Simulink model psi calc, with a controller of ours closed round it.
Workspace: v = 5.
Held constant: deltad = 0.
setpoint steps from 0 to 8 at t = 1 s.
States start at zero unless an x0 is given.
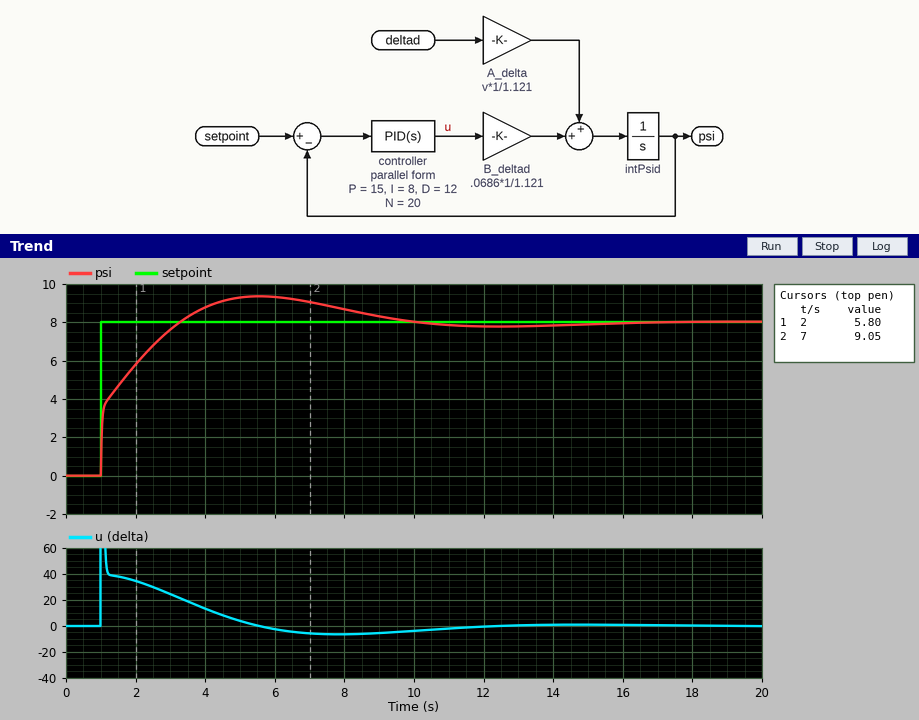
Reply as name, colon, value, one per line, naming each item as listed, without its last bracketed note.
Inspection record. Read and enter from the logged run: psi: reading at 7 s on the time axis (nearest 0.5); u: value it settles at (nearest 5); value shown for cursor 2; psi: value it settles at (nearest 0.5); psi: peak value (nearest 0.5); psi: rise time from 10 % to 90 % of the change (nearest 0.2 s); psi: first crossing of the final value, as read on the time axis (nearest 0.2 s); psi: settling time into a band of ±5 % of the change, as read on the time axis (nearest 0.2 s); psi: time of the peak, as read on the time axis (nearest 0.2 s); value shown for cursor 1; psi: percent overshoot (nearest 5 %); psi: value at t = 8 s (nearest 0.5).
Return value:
psi: reading at 7 s on the time axis: 9.0
u: value it settles at: 0
value shown for cursor 2: 9.05
psi: value it settles at: 8.0
psi: peak value: 9.5
psi: rise time from 10 % to 90 % of the change: 1.8 s
psi: first crossing of the final value, as read on the time axis: 3.2 s
psi: settling time into a band of ±5 % of the change, as read on the time axis: 8.8 s
psi: time of the peak, as read on the time axis: 5.6 s
value shown for cursor 1: 5.80
psi: percent overshoot: 15 %
psi: value at t = 8 s: 8.5
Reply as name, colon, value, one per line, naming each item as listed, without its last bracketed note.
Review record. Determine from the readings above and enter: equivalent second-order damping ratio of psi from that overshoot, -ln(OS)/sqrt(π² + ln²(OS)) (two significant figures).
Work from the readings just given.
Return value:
equivalent second-order damping ratio of psi from that overshoot, -ln(OS)/sqrt(π² + ln²(OS)): 0.52
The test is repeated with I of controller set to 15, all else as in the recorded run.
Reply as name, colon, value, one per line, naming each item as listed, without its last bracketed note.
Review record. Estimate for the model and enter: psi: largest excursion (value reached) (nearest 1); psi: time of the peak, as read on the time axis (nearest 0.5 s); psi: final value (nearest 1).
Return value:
psi: largest excursion (value reached): 10
psi: time of the peak, as read on the time axis: 4.5 s
psi: final value: 8
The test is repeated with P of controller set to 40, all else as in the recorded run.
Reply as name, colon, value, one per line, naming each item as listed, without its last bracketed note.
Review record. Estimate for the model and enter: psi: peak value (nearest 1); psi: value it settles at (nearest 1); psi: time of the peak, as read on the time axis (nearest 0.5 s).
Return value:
psi: peak value: 8
psi: value it settles at: 8
psi: time of the peak, as read on the time axis: 4.5 s
